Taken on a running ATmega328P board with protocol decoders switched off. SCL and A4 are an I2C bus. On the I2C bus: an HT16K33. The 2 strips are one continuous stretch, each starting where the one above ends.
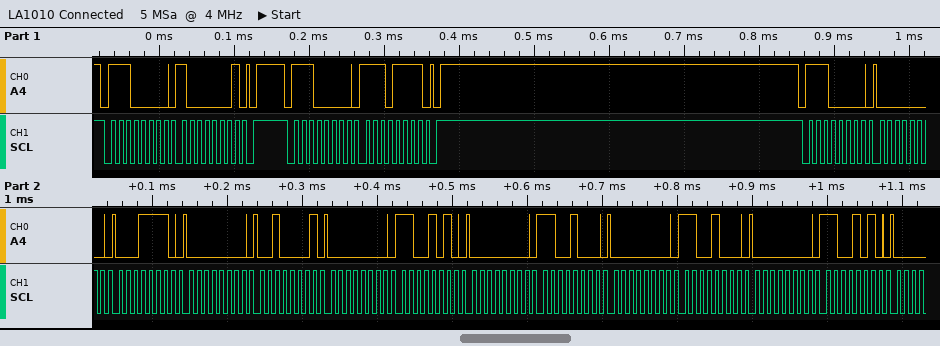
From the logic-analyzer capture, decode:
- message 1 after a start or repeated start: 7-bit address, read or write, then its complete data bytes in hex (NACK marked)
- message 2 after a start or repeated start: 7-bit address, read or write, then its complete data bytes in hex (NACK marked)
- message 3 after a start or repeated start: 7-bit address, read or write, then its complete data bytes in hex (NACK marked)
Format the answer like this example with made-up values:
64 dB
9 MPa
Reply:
0x70 write: 81
0x70 write: EF
0x70 write: 00 1E 00 21 00 CA 00 C8 00 C8 00 CA
